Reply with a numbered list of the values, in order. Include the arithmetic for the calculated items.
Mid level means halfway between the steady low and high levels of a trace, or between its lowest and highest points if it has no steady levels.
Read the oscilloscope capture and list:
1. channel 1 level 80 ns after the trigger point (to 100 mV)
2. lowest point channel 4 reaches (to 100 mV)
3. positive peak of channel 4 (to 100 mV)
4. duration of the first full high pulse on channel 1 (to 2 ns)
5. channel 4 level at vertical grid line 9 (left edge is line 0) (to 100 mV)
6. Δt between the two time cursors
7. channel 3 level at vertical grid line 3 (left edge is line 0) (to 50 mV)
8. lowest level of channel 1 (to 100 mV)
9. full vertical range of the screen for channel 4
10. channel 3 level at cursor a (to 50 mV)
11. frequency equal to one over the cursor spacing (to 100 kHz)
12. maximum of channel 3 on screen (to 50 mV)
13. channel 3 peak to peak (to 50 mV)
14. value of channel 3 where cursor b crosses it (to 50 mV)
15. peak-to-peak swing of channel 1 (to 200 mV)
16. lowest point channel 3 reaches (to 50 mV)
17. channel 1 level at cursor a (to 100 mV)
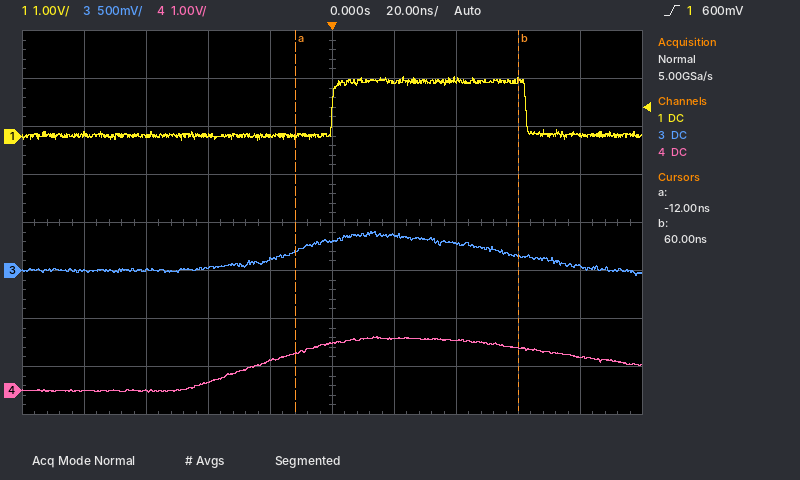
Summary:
1. 0.0 V
2. 0.0 V
3. 1.1 V
4. 62 ns
5. 700 mV
6. 60 ns − (-12 ns) = 72 ns
7. 50 mV
8. -100 mV
9. 8 V
10. 200 mV
11. 1 / 72 ns ≈ 13.9 MHz
12. 400 mV
13. 400 mV − (-50 mV) = 450 mV
14. 150 mV
15. 1.4 V
16. -50 mV
17. 0.0 V
